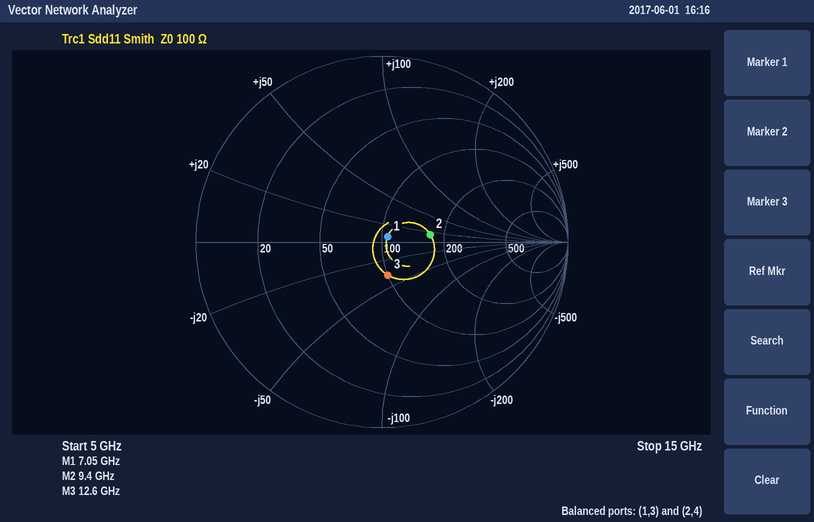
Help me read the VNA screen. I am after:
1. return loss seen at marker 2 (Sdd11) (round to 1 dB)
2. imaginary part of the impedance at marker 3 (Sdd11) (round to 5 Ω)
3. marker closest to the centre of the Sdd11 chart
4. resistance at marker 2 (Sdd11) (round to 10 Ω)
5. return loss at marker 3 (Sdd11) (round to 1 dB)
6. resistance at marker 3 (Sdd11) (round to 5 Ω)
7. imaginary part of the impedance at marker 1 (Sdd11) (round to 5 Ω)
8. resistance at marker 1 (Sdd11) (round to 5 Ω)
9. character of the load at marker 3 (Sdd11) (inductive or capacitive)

12 dB
-35 Ω
marker 1
170 Ω
15 dB
100 Ω
+5 Ω
105 Ω
capacitive
